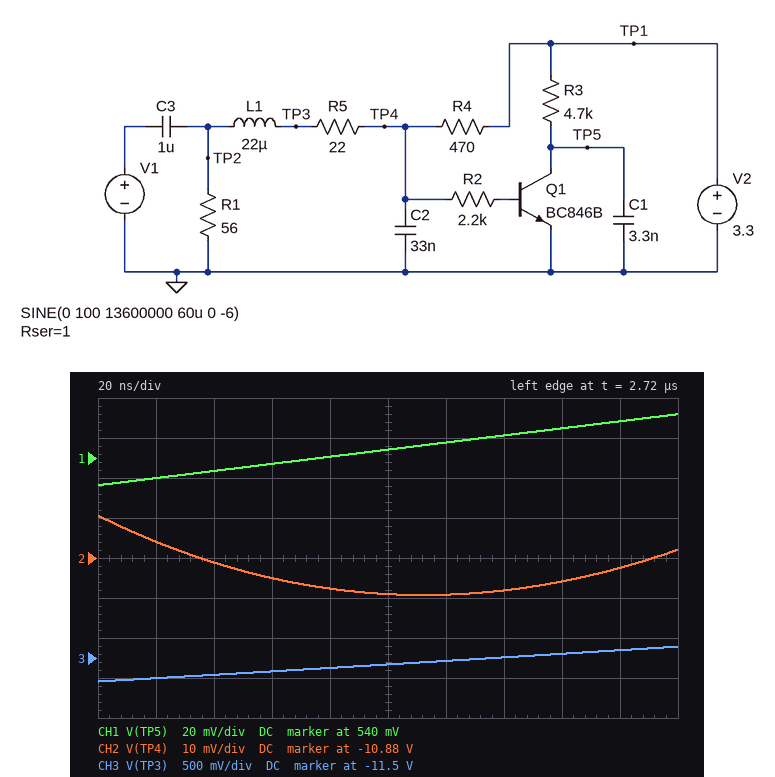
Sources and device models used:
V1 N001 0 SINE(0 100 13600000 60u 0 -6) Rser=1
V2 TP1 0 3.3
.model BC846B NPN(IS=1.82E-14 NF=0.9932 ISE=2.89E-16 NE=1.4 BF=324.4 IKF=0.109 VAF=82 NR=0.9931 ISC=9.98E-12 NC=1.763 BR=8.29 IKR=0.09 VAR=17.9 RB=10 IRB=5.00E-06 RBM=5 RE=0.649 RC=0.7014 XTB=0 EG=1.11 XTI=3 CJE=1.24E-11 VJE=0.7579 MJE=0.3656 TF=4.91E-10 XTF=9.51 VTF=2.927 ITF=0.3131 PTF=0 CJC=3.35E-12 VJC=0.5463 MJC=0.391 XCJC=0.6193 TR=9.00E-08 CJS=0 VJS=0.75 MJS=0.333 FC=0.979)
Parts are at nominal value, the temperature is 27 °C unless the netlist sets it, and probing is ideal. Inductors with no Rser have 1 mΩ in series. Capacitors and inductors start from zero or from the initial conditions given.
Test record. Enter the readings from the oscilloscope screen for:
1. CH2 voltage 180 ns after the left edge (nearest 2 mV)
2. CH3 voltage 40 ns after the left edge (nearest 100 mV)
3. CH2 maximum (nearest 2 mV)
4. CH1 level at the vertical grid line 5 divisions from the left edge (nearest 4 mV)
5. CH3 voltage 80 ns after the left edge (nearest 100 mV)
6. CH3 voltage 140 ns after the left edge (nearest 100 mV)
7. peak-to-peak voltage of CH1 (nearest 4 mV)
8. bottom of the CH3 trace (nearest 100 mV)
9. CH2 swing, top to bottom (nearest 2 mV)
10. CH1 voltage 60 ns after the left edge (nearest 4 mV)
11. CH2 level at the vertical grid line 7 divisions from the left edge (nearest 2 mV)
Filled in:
-10.882 V
-11.7 V
-10.870 V
544 mV
-11.6 V
-11.5 V
36 mV
-11.8 V
20 mV
536 mV
-10.888 V
